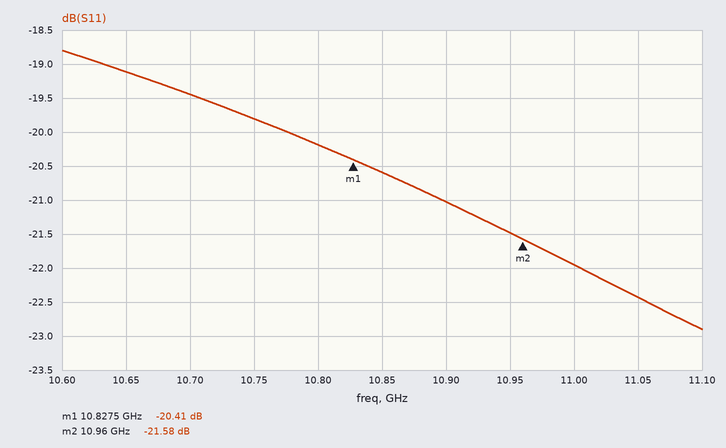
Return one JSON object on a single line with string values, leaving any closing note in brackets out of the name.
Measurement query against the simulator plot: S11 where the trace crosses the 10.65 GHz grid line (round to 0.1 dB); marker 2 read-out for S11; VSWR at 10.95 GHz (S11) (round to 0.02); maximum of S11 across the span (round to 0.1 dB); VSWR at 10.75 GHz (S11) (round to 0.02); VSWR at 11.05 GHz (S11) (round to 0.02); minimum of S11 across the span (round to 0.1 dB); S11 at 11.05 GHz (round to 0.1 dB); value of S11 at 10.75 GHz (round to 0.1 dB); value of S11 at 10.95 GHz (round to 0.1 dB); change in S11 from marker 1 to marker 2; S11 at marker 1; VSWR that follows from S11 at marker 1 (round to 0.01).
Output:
{"S11 where the trace crosses the 10.65 GHz grid line": "-19.1 dB", "marker 2 read-out for S11": "-21.58 dB", "VSWR at 10.95 GHz (S11)": "1.18", "maximum of S11 across the span": "-18.8 dB", "VSWR at 10.75 GHz (S11)": "1.22", "VSWR at 11.05 GHz (S11)": "1.16", "minimum of S11 across the span": "-22.9 dB", "S11 at 11.05 GHz": "-22.4 dB", "value of S11 at 10.75 GHz": "-19.8 dB", "value of S11 at 10.95 GHz": "-21.5 dB", "change in S11 from marker 1 to marker 2": "-1.17 dB", "S11 at marker 1": "-20.41 dB", "VSWR that follows from S11 at marker 1": "1.21"}
